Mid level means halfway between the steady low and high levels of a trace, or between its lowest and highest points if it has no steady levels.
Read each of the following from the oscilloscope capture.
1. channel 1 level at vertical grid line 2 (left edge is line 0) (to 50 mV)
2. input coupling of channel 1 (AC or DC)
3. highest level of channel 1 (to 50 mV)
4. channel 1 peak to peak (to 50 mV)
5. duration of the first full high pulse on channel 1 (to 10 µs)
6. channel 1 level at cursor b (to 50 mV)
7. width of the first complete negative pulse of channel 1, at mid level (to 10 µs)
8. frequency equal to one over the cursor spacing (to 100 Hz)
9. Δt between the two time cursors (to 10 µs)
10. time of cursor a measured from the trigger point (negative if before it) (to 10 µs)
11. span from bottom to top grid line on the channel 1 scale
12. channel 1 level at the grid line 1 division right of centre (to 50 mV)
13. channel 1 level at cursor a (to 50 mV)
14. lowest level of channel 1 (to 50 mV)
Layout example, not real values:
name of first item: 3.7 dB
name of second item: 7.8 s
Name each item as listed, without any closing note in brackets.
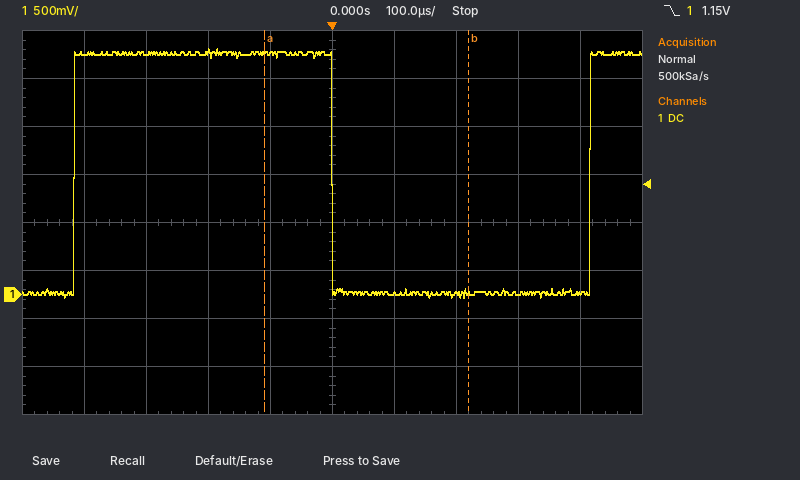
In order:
channel 1 level at vertical grid line 2 (left edge is line 0): 2.50 V
input coupling of channel 1: DC
highest level of channel 1: 2.55 V
channel 1 peak to peak: 2.60 V
duration of the first full high pulse on channel 1: 420 µs
channel 1 level at cursor b: 50 mV
width of the first complete negative pulse of channel 1, at mid level: 420 µs
frequency equal to one over the cursor spacing: 3.0 kHz
Δt between the two time cursors: 330 µs
time of cursor a measured from the trigger point (negative if before it): -110 µs
span from bottom to top grid line on the channel 1 scale: 4 V
channel 1 level at the grid line 1 division right of centre: 0 mV
channel 1 level at cursor a: 2.50 V
lowest level of channel 1: -50 mV
